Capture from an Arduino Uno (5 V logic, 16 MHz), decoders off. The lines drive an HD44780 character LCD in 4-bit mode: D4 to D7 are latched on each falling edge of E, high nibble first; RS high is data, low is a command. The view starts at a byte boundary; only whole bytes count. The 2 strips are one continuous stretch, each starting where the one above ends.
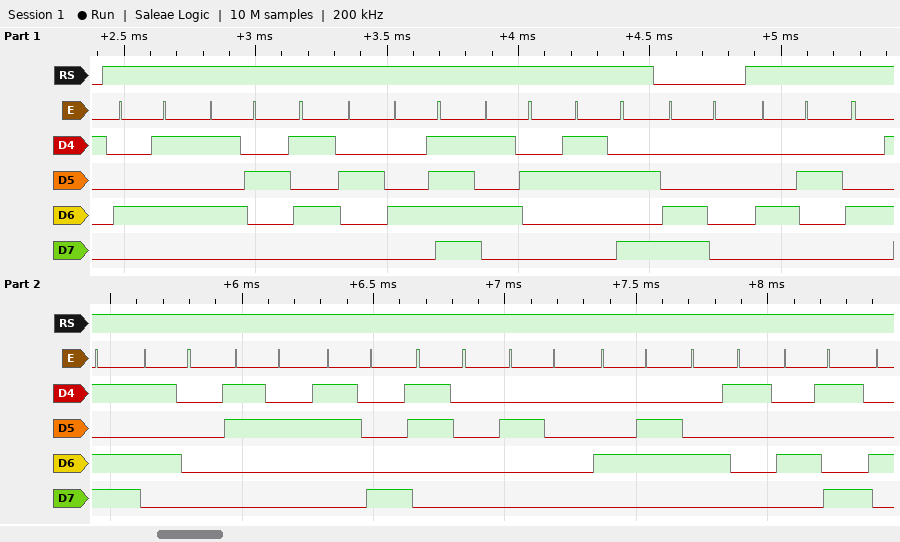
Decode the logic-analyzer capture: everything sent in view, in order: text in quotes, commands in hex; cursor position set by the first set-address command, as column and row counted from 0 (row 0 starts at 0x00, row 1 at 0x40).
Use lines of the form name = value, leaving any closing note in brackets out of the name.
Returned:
everything sent in view, in order: text in quotes, commands in hex = "ERROR:" 0xC0 "BMP280 FAI"
cursor position set by the first set-address command, as column and row counted from 0 = column 0, row 1
